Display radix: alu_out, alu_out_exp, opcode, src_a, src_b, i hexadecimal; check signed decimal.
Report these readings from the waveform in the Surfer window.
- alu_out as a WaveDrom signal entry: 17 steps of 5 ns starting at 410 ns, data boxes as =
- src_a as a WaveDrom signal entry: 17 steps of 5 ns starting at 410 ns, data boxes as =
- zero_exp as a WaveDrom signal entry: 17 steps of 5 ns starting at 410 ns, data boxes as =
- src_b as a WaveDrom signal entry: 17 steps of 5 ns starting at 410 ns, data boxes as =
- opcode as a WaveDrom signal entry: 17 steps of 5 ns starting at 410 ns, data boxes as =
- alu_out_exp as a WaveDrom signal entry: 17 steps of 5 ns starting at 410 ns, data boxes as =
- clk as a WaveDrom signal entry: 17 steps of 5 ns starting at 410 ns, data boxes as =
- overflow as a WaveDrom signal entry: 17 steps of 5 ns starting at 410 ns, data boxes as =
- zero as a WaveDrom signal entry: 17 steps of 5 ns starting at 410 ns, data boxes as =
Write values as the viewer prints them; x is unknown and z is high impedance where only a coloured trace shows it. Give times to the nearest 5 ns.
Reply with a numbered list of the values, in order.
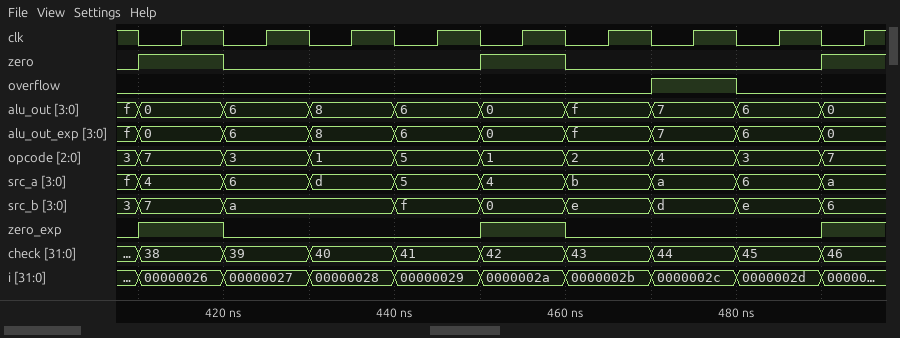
1. {name: 'alu_out', wave: '=.=.=.=.=.=.=.=.=', data: '0 6 8 6 0 f 7 6 0'}
2. {name: 'src_a', wave: '=.=.=.=.=.=.=.=.=', data: '4 6 d 5 4 b a 6 a'}
3. {name: 'zero_exp', wave: '1.0.....1.0.....1'}
4. {name: 'src_b', wave: '=.=...=.=.=.=.=.=', data: '7 a f 0 e d e 6'}
5. {name: 'opcode', wave: '=.=.=.=.=.=.=.=.=', data: '7 3 1 5 1 2 4 3 7'}
6. {name: 'alu_out_exp', wave: '=.=.=.=.=.=.=.=.=', data: '0 6 8 6 0 f 7 6 0'}
7. {name: 'clk', wave: '01010101010101010'}
8. {name: 'overflow', wave: '0...........1.0..'}
9. {name: 'zero', wave: '1.0.....1.0.....1'}
